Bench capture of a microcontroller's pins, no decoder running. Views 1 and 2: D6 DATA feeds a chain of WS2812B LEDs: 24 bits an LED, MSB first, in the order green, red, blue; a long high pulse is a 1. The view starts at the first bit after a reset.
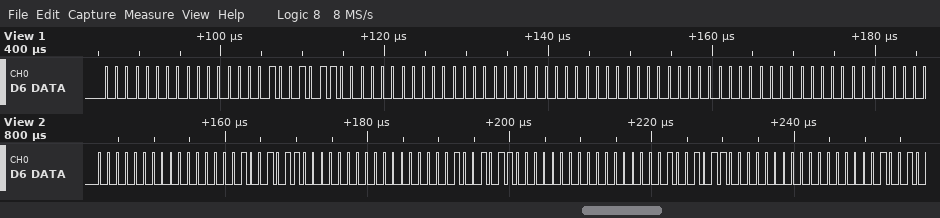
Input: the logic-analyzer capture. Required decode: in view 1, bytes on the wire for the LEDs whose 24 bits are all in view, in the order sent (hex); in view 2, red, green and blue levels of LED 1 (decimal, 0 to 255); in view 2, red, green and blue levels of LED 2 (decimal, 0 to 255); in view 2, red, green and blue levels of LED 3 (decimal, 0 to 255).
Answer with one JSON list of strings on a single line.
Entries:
["00 00 96 00 00 00 00 00 00", "0, 0, 150", "0, 0, 150", "0, 0, 150"]
